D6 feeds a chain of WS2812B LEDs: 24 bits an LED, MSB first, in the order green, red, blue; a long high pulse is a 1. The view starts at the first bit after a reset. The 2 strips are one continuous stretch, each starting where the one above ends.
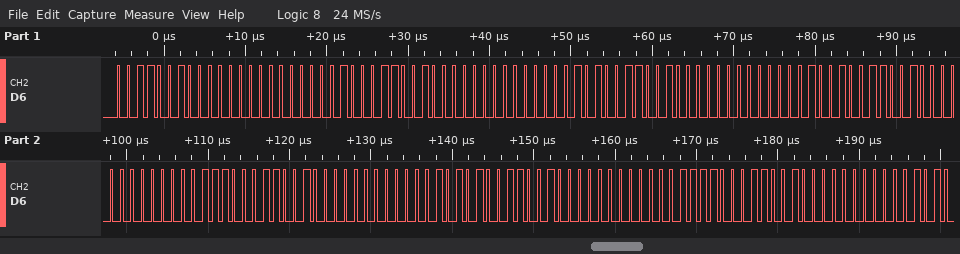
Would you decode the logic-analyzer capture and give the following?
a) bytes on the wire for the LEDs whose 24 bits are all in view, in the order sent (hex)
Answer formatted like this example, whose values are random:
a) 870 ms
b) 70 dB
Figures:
a) 32 00 02 32 00 05 32 00 09 32 00 0E 32 00 15 32 00 1E
